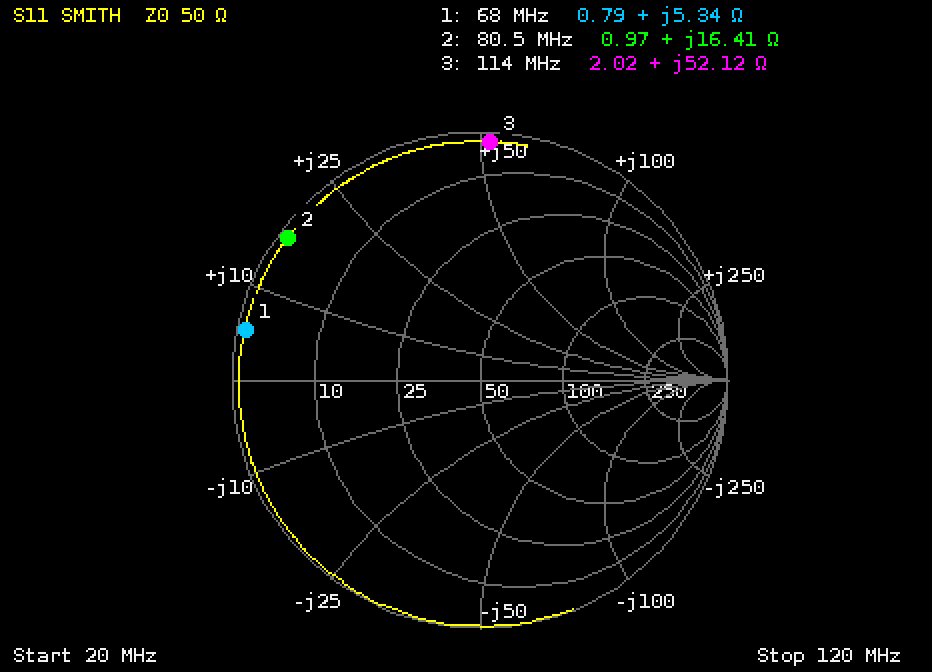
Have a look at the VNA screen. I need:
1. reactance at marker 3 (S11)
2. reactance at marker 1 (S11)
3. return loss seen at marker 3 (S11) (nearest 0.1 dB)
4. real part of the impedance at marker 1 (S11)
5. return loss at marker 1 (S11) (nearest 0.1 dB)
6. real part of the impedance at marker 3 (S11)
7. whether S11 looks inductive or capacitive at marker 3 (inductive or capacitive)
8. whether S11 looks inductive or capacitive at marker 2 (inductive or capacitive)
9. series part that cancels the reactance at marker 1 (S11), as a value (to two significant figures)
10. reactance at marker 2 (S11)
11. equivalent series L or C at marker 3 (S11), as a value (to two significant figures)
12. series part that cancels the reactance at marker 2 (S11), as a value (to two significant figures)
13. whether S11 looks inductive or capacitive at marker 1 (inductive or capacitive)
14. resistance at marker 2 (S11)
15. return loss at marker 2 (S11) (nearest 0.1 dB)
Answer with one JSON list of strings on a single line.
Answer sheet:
["+52.12 Ω", "+5.34 Ω", "0.3 dB", "0.79 Ω", "0.3 dB", "2.02 Ω", "inductive", "inductive", "440 pF", "+16.41 Ω", "73 nH", "120 pF", "inductive", "0.97 Ω", "0.3 dB"]
